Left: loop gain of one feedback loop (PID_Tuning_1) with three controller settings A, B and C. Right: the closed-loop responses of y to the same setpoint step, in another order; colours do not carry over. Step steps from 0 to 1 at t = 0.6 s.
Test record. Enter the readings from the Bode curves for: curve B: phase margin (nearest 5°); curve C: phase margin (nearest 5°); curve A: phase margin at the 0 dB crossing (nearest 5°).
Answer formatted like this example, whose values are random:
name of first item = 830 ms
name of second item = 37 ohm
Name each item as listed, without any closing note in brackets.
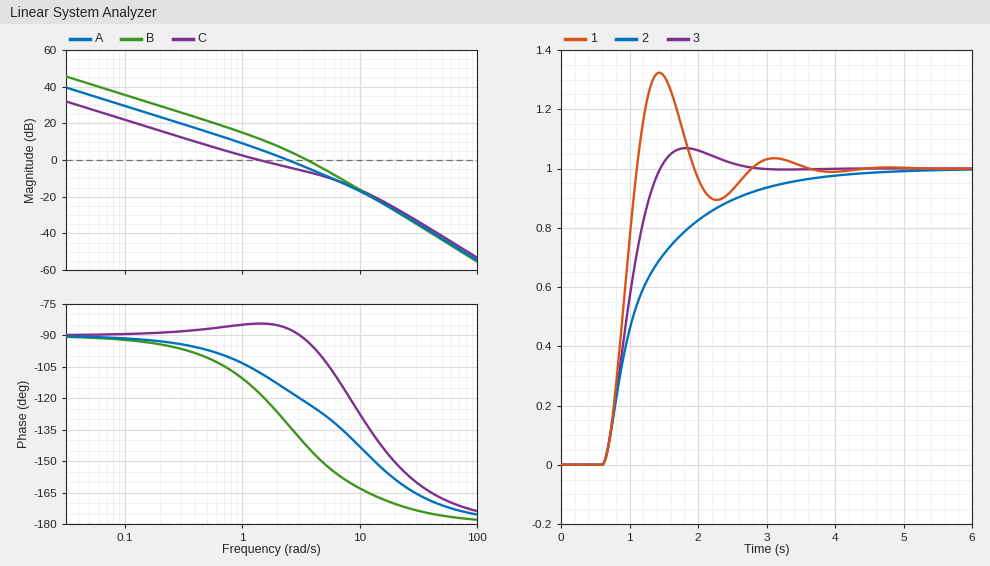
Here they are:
curve B: phase margin = 35°
curve C: phase margin = 95°
curve A: phase margin at the 0 dB crossing = 65°
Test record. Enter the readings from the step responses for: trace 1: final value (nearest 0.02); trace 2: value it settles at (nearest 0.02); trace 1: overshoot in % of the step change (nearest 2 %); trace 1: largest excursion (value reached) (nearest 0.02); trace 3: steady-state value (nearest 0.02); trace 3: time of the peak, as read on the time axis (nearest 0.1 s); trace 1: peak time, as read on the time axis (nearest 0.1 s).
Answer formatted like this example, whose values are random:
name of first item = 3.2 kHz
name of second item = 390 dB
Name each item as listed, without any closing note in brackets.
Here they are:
trace 1: final value = 1.00
trace 2: value it settles at = 1.00
trace 1: overshoot in % of the step change = 32 %
trace 1: largest excursion (value reached) = 1.32
trace 3: steady-state value = 1.00
trace 3: time of the peak, as read on the time axis = 1.8 s
trace 1: peak time, as read on the time axis = 1.4 s
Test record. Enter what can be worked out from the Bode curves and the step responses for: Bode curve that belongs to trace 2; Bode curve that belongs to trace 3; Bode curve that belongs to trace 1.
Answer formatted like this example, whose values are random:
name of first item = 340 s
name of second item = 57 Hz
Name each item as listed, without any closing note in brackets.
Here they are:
Bode curve that belongs to trace 2 = C
Bode curve that belongs to trace 3 = A
Bode curve that belongs to trace 1 = B
